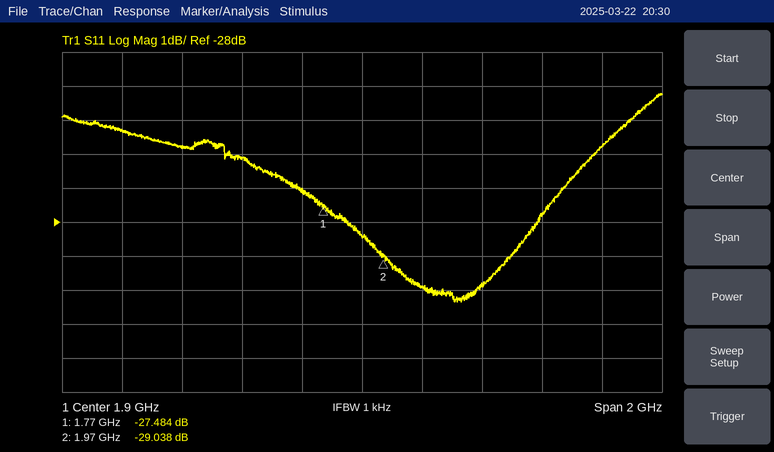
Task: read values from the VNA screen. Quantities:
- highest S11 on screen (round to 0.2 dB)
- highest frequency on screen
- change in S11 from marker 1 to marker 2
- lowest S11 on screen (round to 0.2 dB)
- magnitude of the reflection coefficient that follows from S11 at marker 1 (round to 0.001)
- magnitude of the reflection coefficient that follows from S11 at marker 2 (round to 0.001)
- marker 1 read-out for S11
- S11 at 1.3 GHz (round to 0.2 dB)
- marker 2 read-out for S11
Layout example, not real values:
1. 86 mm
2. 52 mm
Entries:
1. -24.2 dB
2. 2.9 GHz
3. -1.554 dB
4. -30.4 dB
5. 0.042
6. 0.035
7. -27.484 dB
8. -25.8 dB
9. -29.038 dB
